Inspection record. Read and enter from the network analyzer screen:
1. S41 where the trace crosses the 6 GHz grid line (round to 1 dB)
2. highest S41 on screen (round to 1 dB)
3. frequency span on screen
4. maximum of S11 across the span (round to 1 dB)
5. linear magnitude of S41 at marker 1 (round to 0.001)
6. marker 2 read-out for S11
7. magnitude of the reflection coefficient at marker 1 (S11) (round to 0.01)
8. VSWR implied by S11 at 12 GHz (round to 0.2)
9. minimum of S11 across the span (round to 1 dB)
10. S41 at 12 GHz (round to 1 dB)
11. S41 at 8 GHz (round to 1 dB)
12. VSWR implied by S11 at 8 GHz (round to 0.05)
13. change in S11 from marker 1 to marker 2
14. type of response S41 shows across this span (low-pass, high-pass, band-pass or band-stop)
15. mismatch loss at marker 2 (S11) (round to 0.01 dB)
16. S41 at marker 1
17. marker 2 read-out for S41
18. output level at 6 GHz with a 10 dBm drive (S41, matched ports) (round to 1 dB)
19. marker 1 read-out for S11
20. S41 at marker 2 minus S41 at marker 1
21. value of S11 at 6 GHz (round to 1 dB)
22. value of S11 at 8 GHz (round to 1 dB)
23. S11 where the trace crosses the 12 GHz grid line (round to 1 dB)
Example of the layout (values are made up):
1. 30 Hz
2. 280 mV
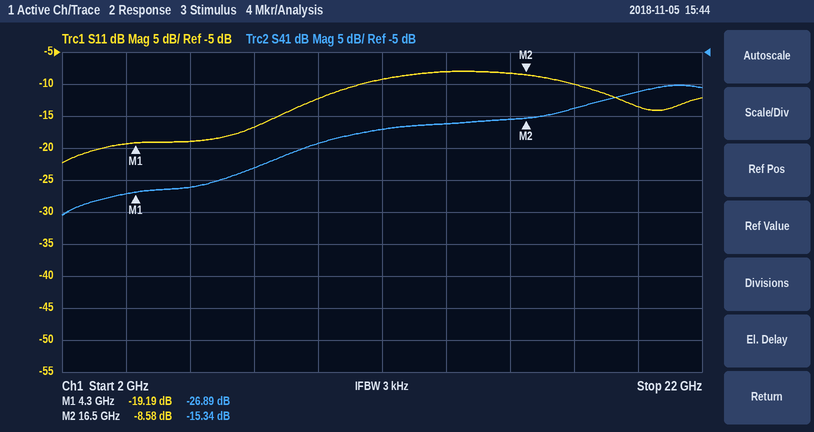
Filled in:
1. -26 dB
2. -10 dB
3. 20 GHz
4. -8 dB
5. 0.045
6. -8.58 dB
7. 0.11
8. 2.0
9. -22 dB
10. -17 dB
11. -23 dB
12. 1.35
13. 10.61 dB
14. high-pass
15. 0.65 dB
16. -26.89 dB
17. -15.34 dB
18. -16 dBm
19. -19.19 dB
20. 11.55 dB
21. -19 dB
22. -17 dB
23. -9 dB
